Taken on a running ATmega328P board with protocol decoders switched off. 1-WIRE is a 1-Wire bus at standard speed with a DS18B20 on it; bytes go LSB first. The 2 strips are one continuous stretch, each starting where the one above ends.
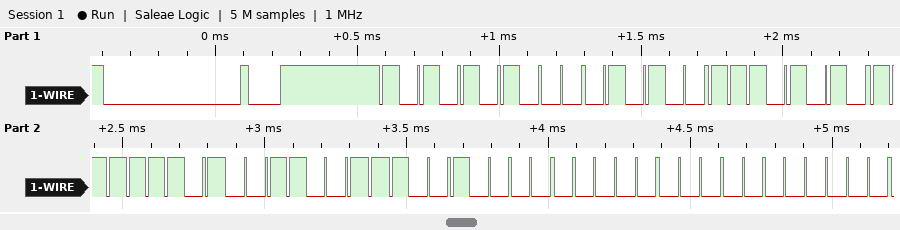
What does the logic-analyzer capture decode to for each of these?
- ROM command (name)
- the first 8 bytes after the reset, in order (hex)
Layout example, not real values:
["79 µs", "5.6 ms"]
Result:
["Match ROM", "55 28 57 BF CC 09 00 00"]
